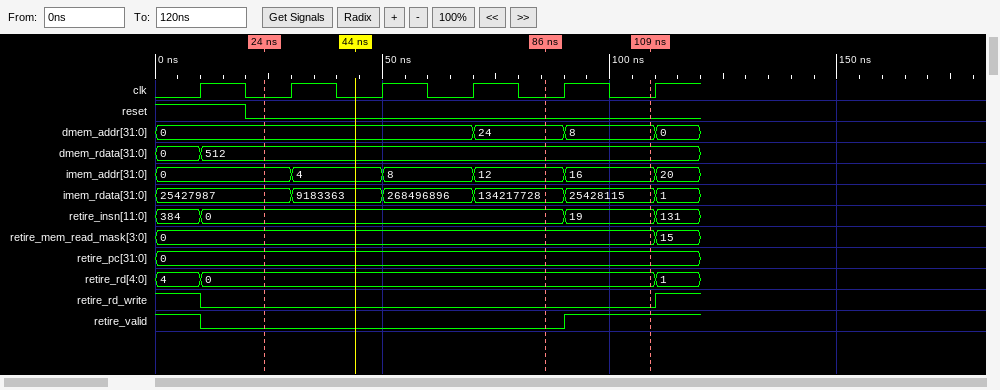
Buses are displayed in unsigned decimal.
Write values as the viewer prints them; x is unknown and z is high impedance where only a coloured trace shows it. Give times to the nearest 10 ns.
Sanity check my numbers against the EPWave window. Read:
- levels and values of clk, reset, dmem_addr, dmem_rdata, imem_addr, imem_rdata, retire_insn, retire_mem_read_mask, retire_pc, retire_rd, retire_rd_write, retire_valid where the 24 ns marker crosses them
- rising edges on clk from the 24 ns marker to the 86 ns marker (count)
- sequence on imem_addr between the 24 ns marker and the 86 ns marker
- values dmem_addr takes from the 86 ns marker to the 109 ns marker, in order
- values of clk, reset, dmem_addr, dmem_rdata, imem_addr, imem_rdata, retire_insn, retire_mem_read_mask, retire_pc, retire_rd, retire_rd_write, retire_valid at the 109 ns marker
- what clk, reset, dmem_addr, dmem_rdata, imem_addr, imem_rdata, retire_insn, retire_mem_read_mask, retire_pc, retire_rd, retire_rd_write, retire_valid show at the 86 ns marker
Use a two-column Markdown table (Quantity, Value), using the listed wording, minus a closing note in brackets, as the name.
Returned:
| Quantity | Value |
|---|---|
| levels and values of clk, reset, dmem_addr, dmem_rdata, imem_addr, imem_rdata, retire_insn, retire_mem_read_mask, retire_pc, retire_rd, retire_rd_write, retire_valid where the 24 ns marker crosses them | clk=0, reset=0, dmem_addr=0, dmem_rdata=512, imem_addr=0, imem_rdata=25427987, retire_insn=0, retire_mem_read_mask=0, retire_pc=0, retire_rd=0, retire_rd_write=0, retire_valid=0 |
| rising edges on clk from the 24 ns marker to the 86 ns marker | 3 |
| sequence on imem_addr between the 24 ns marker and the 86 ns marker | 0, 4, 8, 12 |
| values dmem_addr takes from the 86 ns marker to the 109 ns marker, in order | 24, 8 |
| values of clk, reset, dmem_addr, dmem_rdata, imem_addr, imem_rdata, retire_insn, retire_mem_read_mask, retire_pc, retire_rd, retire_rd_write, retire_valid at the 109 ns marker | clk=0, reset=0, dmem_addr=8, dmem_rdata=512, imem_addr=16, imem_rdata=25428115, retire_insn=19, retire_mem_read_mask=0, retire_pc=0, retire_rd=0, retire_rd_write=0, retire_valid=1 |
| what clk, reset, dmem_addr, dmem_rdata, imem_addr, imem_rdata, retire_insn, retire_mem_read_mask, retire_pc, retire_rd, retire_rd_write, retire_valid show at the 86 ns marker | clk=0, reset=0, dmem_addr=24, dmem_rdata=512, imem_addr=12, imem_rdata=134217728, retire_insn=0, retire_mem_read_mask=0, retire_pc=0, retire_rd=0, retire_rd_write=0, retire_valid=0 |
